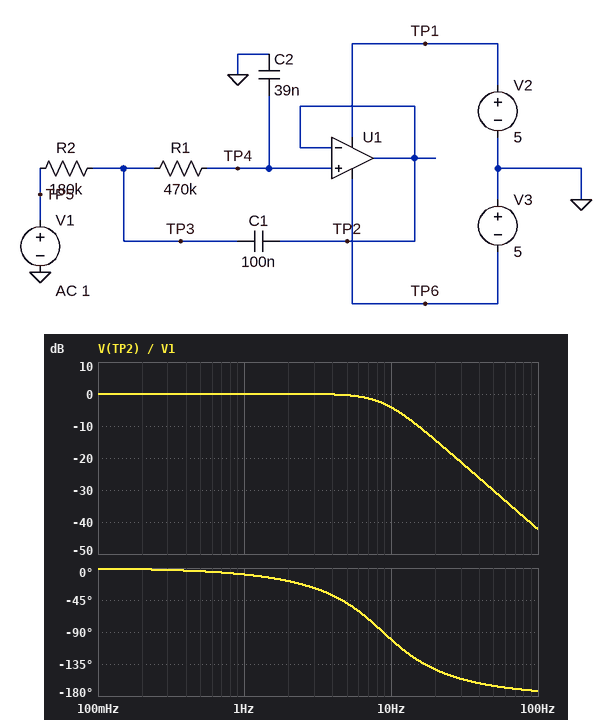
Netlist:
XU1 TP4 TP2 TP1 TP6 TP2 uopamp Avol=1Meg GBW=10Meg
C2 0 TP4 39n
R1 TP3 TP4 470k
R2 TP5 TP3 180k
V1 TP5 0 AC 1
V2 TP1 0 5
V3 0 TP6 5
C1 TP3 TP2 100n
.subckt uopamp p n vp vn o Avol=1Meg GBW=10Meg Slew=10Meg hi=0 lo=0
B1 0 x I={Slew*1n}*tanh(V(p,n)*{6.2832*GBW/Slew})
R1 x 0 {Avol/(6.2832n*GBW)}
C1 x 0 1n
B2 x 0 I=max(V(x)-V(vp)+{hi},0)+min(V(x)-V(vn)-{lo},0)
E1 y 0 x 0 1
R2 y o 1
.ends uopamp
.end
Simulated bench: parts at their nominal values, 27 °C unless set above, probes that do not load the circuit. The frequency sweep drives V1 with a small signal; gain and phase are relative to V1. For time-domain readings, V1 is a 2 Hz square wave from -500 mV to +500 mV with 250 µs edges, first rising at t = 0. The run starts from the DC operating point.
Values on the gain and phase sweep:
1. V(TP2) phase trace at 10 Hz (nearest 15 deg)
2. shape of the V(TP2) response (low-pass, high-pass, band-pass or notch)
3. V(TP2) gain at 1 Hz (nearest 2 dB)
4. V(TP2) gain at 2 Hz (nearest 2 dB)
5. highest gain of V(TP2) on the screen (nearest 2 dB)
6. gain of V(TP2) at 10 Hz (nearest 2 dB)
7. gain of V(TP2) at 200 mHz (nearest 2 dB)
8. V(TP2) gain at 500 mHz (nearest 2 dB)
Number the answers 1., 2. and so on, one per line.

1. -105 deg
2. low-pass
3. 0 dB
4. 0 dB
5. 0 dB
6. -4 dB
7. 0 dB
8. 0 dB
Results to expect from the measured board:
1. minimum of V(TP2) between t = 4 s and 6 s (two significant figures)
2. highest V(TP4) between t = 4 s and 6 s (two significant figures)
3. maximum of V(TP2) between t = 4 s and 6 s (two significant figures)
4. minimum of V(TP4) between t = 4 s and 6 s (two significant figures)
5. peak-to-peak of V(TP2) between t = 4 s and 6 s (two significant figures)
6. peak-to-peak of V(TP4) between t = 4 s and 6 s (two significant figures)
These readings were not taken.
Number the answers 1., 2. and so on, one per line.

1. -550 mV
2. 550 mV
3. 550 mV
4. -550 mV
5. 1.1 V
6. 1.1 V
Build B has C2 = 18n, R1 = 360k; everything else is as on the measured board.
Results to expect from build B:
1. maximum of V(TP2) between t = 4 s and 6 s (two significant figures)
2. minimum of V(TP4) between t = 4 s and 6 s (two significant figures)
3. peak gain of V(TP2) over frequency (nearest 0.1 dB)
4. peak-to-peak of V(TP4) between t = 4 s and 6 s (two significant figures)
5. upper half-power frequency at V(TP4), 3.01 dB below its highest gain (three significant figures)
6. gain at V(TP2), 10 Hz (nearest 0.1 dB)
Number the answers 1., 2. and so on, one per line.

1. 710 mV
2. -710 mV
3. 1.9 dB
4. 1.4 V
5. 17.4 Hz
6. 1.8 dB
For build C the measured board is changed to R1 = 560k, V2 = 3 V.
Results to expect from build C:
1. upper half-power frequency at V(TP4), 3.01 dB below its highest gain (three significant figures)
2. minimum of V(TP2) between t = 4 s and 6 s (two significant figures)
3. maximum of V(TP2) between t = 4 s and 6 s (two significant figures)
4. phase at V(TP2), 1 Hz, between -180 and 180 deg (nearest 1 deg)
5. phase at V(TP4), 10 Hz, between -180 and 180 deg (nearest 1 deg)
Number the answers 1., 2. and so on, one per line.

1. 7.79 Hz
2. -540 mV
3. 540 mV
4. -10 deg
5. -107 deg
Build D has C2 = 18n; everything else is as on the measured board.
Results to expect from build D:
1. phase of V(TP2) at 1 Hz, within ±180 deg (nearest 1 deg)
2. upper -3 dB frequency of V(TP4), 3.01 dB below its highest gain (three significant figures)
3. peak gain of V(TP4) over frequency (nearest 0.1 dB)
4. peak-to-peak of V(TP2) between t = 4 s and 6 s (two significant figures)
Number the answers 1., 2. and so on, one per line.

1. -4 deg
2. 15.2 Hz
3. 1.6 dB
4. 1.4 V
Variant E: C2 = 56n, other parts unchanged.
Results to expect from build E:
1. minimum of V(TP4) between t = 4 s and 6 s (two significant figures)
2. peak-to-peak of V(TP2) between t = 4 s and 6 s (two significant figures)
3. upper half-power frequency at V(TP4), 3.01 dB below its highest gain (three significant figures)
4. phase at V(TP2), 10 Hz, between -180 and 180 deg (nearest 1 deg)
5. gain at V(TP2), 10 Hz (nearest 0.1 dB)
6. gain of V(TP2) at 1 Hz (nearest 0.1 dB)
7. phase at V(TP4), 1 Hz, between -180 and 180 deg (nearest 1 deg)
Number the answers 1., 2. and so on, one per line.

1. -510 mV
2. 1.0 V
3. 6.02 Hz
4. -111 deg
5. -7.8 dB
6. -0.1 dB
7. -13 deg
